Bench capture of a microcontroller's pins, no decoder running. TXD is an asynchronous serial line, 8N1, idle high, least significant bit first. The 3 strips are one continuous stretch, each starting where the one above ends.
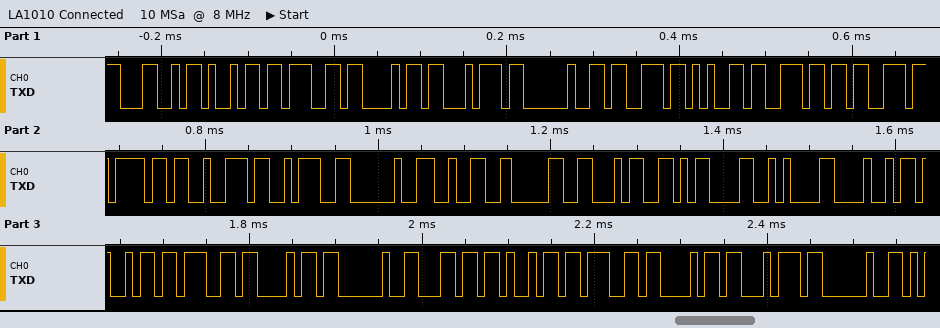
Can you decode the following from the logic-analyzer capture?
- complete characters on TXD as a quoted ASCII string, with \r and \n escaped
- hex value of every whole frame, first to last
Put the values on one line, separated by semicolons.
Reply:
"Light sensor: 204\r\nHigh light "; 4C 69 67 68 74 20 73 65 6E 73 6F 72 3A 20 32 30 34 0D 0A 48 69 67 68 20 6C 69 67 68 74 20
